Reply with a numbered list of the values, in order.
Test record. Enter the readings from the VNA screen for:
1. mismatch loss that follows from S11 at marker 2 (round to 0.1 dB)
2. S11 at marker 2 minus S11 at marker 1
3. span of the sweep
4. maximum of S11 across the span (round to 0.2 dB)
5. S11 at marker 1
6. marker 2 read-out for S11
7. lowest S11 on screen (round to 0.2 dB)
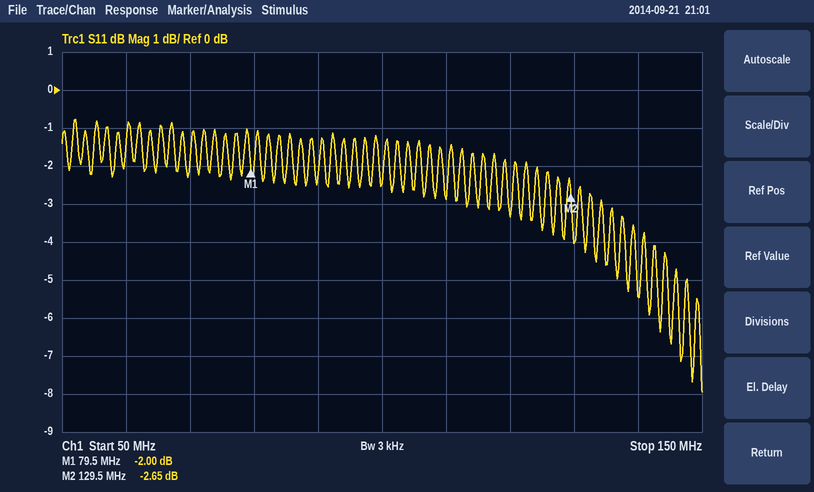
1. 3.4 dB
2. -0.65 dB
3. 100 MHz
4. -0.8 dB
5. -2.00 dB
6. -2.65 dB
7. -8.0 dB
